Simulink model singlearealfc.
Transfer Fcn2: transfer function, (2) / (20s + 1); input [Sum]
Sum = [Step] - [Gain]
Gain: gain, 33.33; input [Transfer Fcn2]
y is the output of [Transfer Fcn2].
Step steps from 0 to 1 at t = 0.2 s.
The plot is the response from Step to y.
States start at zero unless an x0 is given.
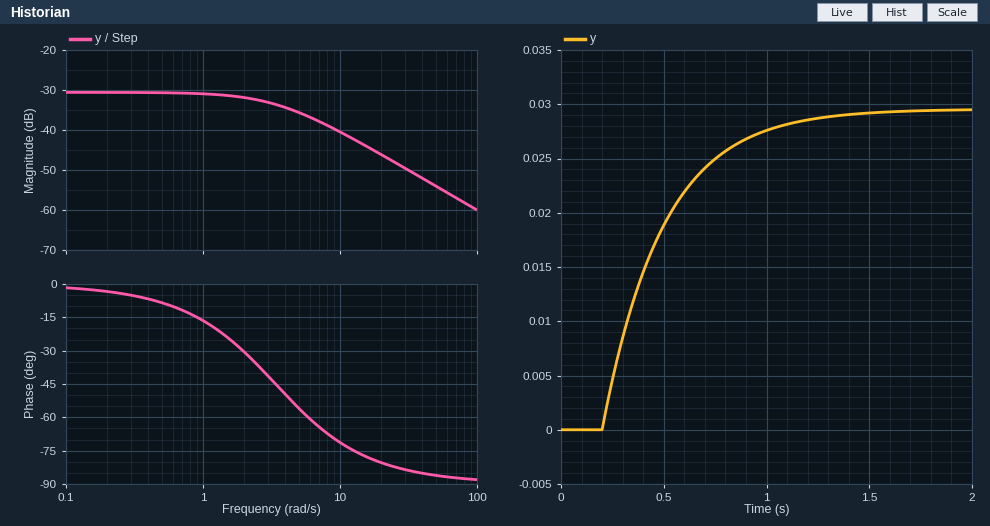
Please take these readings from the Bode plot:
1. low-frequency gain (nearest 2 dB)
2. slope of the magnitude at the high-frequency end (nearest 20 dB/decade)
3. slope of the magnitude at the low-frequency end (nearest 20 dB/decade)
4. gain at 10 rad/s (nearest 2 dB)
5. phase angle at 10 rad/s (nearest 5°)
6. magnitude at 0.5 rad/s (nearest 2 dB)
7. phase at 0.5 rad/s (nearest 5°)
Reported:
-30 dB
-20 dB/decade
0 dB/decade
-40 dB
-70°
-30 dB
-10°
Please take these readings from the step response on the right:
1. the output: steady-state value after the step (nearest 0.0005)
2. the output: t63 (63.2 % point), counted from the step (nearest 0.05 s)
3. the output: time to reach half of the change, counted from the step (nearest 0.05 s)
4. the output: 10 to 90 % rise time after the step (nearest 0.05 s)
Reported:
0.0295
0.30 s
0.20 s
0.65 s
